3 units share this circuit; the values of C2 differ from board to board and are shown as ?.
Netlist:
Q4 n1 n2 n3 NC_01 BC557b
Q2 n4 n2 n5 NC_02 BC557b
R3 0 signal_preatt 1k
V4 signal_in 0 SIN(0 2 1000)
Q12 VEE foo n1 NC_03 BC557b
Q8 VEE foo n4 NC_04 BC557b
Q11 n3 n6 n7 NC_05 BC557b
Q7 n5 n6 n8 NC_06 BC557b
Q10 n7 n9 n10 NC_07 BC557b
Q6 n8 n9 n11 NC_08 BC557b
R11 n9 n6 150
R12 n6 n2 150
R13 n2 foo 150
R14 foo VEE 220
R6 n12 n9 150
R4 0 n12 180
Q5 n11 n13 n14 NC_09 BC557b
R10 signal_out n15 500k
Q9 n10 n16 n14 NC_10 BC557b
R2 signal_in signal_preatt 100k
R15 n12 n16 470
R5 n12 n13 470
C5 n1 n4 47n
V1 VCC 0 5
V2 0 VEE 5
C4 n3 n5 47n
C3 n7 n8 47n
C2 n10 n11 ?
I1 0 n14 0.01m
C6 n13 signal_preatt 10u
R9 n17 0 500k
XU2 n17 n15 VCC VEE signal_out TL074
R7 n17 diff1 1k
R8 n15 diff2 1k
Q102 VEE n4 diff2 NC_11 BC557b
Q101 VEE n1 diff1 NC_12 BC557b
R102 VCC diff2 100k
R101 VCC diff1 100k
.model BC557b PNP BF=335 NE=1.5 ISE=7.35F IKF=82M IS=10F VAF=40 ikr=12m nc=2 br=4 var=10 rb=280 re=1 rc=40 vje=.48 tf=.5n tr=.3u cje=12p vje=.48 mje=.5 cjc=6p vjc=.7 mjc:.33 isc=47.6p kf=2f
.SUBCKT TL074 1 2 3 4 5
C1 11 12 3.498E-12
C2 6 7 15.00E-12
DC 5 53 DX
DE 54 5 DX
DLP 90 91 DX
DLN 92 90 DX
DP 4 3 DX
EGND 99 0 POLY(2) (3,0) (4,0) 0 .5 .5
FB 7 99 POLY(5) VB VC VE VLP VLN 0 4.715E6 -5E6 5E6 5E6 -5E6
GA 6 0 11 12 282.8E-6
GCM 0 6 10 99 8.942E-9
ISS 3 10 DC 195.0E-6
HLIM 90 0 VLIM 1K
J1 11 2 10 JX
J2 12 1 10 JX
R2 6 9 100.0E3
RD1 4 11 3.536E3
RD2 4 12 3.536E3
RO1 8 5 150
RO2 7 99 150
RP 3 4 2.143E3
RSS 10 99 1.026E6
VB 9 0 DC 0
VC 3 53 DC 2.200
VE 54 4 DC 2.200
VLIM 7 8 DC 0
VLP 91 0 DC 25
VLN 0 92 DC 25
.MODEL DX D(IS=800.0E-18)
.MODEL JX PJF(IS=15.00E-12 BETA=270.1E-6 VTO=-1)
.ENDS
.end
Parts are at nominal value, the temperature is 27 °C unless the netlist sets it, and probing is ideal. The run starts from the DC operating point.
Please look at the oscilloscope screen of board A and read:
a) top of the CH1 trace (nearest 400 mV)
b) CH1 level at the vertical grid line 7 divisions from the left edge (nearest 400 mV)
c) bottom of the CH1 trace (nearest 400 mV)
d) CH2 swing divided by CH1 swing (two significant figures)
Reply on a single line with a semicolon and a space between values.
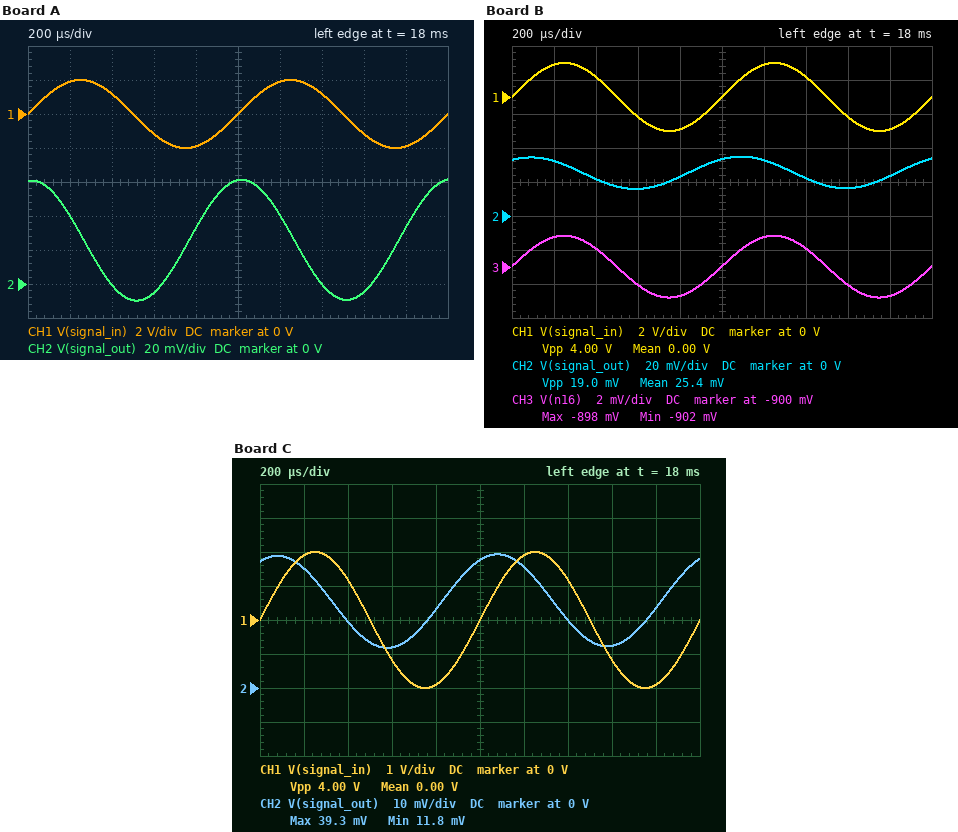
2.0 V; 1.2 V; -2.0 V; 0.018
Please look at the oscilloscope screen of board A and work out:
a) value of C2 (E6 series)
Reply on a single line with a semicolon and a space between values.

22 nF
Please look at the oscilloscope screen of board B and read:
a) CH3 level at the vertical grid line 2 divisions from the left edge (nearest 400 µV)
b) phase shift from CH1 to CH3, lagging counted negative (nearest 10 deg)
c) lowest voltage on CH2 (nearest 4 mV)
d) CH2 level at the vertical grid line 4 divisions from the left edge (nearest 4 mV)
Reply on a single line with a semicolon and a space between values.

-898.8 mV; 0 deg; 16 mV; 24 mV
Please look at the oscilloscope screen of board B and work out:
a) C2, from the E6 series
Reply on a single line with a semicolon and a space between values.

100 nF
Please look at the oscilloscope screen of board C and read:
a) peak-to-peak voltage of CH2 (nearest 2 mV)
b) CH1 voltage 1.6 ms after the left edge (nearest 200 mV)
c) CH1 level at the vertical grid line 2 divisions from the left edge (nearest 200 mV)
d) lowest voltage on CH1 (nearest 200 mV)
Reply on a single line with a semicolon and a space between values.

28 mV; -1.2 V; 1.2 V; -2.0 V
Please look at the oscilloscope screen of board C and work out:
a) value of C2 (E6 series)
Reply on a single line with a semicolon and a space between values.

68 nF
